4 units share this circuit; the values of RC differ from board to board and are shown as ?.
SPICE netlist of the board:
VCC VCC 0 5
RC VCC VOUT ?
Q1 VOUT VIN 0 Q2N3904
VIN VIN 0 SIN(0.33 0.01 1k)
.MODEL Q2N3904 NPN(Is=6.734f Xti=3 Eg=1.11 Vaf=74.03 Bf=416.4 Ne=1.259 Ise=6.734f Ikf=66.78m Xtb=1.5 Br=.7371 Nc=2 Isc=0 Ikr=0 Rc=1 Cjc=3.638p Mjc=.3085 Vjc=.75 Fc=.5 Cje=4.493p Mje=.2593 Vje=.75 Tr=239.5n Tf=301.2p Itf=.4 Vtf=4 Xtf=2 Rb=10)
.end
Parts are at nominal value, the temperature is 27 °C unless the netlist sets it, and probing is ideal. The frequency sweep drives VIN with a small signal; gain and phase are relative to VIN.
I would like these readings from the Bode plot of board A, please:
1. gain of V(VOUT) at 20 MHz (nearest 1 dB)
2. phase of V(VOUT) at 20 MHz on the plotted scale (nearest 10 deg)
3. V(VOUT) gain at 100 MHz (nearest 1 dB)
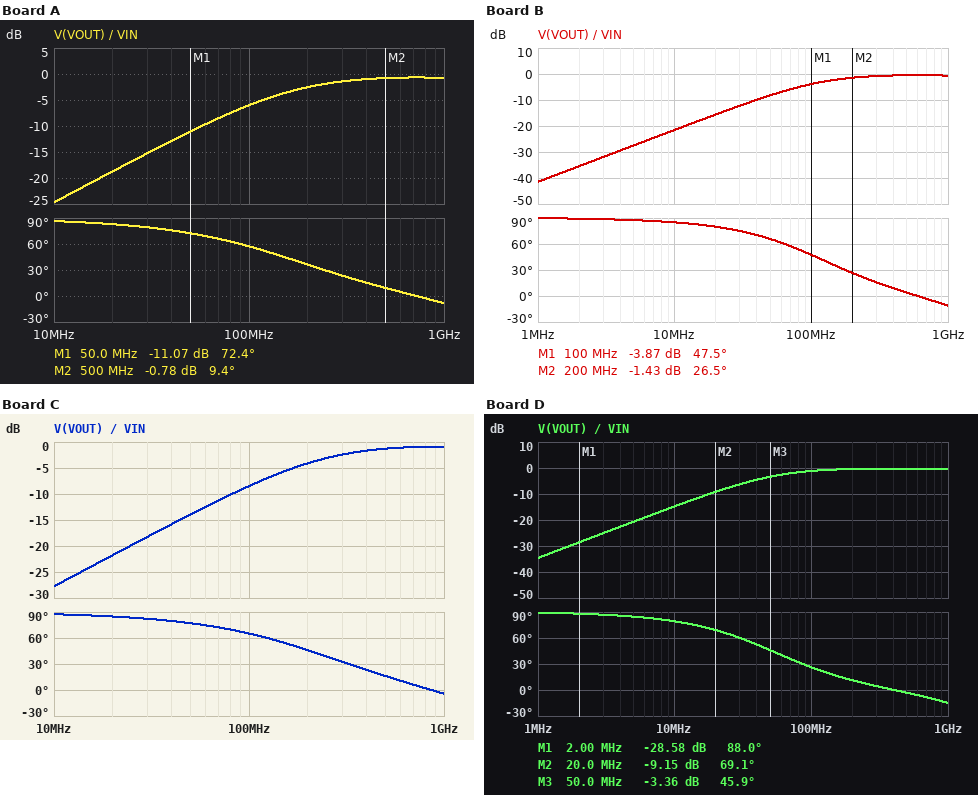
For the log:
-19 dB
80 deg
-6 dB
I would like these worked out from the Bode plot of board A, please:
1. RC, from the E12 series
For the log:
470 Ω
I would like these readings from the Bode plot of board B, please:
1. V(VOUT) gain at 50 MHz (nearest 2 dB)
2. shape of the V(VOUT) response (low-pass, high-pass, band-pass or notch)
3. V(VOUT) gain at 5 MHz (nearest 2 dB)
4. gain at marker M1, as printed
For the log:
-8 dB
high-pass
-28 dB
-3.87 dB
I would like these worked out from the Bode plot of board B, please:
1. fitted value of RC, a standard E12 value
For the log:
680 Ω
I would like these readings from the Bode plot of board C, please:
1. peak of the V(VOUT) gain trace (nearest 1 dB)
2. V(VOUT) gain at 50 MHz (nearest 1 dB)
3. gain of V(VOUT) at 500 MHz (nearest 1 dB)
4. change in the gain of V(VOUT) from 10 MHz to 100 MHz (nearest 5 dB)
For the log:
-1 dB
-14 dB
-1 dB
20 dB
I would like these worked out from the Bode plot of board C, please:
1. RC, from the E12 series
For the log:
330 Ω
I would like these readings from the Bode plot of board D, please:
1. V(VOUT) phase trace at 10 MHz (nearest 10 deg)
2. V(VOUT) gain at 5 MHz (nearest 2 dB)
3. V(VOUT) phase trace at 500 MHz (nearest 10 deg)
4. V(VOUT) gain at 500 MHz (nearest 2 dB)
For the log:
80 deg
-20 dB
0 deg
0 dB
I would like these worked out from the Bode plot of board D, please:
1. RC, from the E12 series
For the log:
1.5 kΩ
